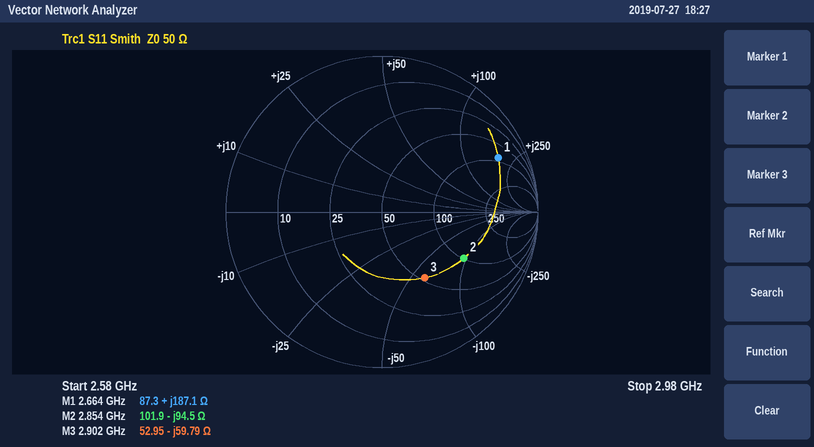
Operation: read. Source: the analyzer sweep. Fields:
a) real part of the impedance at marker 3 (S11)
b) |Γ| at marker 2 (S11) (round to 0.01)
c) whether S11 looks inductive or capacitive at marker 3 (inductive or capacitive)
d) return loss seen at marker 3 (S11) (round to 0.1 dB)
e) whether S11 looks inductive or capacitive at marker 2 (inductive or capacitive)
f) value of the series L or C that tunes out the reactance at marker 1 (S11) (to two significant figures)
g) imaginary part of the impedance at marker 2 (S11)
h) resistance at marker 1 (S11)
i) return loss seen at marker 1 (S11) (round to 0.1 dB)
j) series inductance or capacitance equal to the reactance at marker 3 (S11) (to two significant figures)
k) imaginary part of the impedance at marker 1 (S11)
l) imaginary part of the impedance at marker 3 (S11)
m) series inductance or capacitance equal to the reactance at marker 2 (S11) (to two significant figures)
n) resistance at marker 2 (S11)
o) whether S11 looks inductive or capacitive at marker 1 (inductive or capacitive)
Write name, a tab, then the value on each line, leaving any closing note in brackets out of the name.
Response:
real part of the impedance at marker 3	52.95 Ω
|Γ| at marker 2 (S11)	0.60
whether S11 looks inductive or capacitive at marker 3	capacitive
return loss seen at marker 3 (S11)	6.0 dB
whether S11 looks inductive or capacitive at marker 2	capacitive
value of the series L or C that tunes out the reactance at marker 1 (S11)	320 fF
imaginary part of the impedance at marker 2	-94.5 Ω
resistance at marker 1	87.3 Ω
return loss seen at marker 1 (S11)	1.7 dB
series inductance or capacitance equal to the reactance at marker 3 (S11)	920 fF
imaginary part of the impedance at marker 1	+187.1 Ω
imaginary part of the impedance at marker 3	-59.79 Ω
series inductance or capacitance equal to the reactance at marker 2 (S11)	590 fF
resistance at marker 2	101.9 Ω
whether S11 looks inductive or capacitive at marker 1	inductive
